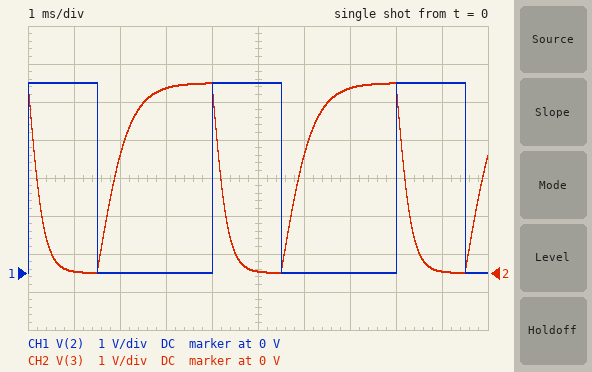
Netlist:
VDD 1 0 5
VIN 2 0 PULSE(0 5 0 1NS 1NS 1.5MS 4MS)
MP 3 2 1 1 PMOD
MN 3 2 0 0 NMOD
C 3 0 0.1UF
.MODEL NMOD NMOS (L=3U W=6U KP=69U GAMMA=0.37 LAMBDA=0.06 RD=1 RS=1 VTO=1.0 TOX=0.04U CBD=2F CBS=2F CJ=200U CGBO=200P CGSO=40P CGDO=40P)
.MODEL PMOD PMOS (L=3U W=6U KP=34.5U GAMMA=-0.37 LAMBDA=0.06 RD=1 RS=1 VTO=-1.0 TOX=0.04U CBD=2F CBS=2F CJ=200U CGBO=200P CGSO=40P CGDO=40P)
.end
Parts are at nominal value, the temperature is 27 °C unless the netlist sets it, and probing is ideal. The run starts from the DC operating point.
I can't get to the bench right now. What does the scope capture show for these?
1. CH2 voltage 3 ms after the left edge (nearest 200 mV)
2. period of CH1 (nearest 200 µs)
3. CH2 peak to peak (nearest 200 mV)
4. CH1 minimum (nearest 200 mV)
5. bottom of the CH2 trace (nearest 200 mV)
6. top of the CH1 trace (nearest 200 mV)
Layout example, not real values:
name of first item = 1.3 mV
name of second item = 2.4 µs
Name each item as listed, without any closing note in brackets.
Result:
CH2 voltage 3 ms after the left edge = 4.8 V
period of CH1 = 4.0 ms
CH2 peak to peak = 5.0 V
CH1 minimum = 0 V
bottom of the CH2 trace = 0 V
top of the CH1 trace = 5.0 V
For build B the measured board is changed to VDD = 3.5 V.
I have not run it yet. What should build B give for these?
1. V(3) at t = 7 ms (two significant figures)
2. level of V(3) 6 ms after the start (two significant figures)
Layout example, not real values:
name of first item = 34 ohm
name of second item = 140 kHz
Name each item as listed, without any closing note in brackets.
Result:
V(3) at t = 7 ms = 2.9 V
level of V(3) 6 ms after the start = 1.3 V
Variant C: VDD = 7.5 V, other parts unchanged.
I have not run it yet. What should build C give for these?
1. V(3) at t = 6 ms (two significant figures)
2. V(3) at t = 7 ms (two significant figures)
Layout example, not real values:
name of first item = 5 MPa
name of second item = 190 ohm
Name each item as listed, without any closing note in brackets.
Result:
V(3) at t = 6 ms = 6.5 V
V(3) at t = 7 ms = 7.5 V
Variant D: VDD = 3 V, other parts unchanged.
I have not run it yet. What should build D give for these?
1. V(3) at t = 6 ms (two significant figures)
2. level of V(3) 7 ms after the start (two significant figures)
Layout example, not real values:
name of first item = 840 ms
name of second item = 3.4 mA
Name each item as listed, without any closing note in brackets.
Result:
V(3) at t = 6 ms = 800 mV
level of V(3) 7 ms after the start = 2.1 V
